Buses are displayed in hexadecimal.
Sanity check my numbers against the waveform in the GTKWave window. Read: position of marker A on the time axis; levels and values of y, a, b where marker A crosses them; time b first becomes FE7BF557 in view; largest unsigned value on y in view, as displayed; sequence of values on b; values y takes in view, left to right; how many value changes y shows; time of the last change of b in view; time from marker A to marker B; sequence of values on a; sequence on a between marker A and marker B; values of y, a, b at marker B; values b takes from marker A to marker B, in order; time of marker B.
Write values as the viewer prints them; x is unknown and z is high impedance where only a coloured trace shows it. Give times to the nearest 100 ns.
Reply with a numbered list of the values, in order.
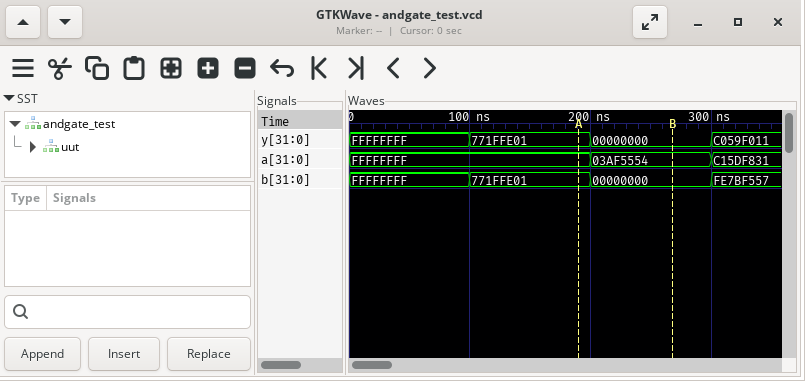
1. 200 ns
2. y=771FFE01, a=FFFFFFFF, b=771FFE01
3. 300 ns
4. FFFFFFFF
5. FFFFFFFF, 771FFE01, 00000000, FE7BF557
6. FFFFFFFF, 771FFE01, 00000000, C059F011
7. 3
8. 300 ns
9. 100 ns
10. FFFFFFFF, 03AF5554, C15DF831
11. FFFFFFFF, 03AF5554
12. y=00000000, a=03AF5554, b=00000000
13. 771FFE01, 00000000
14. 300 ns
